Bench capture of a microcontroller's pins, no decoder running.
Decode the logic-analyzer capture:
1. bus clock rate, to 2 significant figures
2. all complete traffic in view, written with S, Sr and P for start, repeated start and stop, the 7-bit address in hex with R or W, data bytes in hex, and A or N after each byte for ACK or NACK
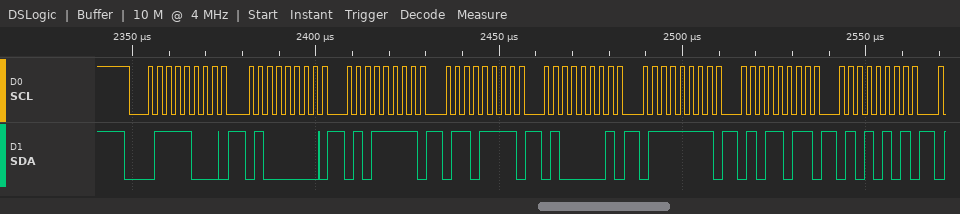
400 kHz
S 3CW A 40 A 5F A 6F A 41 A 7F A 5B A 55 A
